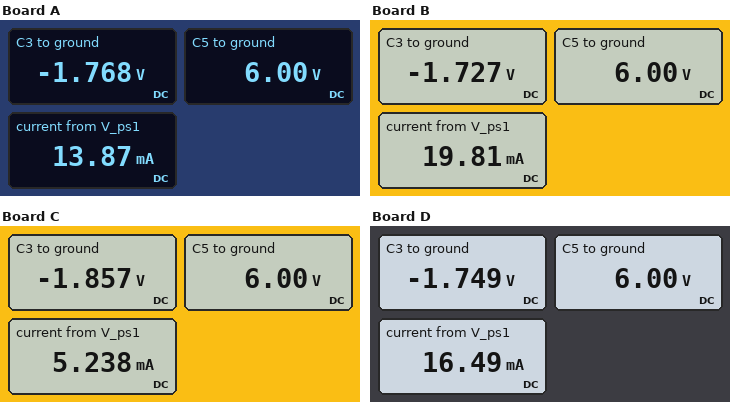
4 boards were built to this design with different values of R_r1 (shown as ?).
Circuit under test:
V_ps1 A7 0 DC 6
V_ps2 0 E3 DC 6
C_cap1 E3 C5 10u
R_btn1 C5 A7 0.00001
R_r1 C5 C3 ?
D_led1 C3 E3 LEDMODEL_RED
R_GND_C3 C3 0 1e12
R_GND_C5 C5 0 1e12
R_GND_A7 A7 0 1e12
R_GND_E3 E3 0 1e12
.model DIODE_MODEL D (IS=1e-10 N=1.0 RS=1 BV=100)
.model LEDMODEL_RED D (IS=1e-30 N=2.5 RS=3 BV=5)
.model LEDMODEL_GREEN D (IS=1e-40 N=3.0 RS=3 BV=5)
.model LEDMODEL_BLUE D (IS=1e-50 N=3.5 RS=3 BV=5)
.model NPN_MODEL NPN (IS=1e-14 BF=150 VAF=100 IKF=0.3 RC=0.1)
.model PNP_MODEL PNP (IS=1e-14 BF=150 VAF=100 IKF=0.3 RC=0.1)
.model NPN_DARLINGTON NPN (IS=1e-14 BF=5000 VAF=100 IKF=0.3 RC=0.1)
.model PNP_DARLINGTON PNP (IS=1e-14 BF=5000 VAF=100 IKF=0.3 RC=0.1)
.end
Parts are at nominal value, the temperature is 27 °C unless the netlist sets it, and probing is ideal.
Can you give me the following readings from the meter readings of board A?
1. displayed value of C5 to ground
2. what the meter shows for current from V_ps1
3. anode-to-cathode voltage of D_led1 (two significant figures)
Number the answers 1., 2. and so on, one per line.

1. 6.00 V
2. 13.87 mA
3. 4.2 V
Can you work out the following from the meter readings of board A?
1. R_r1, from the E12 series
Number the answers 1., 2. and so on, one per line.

1. 560 Ω
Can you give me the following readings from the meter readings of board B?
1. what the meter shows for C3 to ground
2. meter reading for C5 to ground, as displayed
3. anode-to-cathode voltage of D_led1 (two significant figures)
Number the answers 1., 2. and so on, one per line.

1. -1.727 V
2. 6.00 V
3. 4.3 V
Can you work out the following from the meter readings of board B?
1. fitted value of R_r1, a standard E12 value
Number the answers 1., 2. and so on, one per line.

1. 390 Ω
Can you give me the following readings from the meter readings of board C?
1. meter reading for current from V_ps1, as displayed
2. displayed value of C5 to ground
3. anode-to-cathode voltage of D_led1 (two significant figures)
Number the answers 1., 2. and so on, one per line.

1. 5.238 mA
2. 6.00 V
3. 4.1 V
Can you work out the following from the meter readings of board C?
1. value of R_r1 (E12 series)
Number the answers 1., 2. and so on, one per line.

1. 1.5 kΩ
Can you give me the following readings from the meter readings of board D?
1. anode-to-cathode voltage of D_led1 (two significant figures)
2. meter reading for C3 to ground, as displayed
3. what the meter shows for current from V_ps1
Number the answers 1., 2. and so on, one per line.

1. 4.3 V
2. -1.749 V
3. 16.49 mA
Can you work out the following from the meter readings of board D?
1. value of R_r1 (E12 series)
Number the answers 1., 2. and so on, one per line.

1. 470 Ω
